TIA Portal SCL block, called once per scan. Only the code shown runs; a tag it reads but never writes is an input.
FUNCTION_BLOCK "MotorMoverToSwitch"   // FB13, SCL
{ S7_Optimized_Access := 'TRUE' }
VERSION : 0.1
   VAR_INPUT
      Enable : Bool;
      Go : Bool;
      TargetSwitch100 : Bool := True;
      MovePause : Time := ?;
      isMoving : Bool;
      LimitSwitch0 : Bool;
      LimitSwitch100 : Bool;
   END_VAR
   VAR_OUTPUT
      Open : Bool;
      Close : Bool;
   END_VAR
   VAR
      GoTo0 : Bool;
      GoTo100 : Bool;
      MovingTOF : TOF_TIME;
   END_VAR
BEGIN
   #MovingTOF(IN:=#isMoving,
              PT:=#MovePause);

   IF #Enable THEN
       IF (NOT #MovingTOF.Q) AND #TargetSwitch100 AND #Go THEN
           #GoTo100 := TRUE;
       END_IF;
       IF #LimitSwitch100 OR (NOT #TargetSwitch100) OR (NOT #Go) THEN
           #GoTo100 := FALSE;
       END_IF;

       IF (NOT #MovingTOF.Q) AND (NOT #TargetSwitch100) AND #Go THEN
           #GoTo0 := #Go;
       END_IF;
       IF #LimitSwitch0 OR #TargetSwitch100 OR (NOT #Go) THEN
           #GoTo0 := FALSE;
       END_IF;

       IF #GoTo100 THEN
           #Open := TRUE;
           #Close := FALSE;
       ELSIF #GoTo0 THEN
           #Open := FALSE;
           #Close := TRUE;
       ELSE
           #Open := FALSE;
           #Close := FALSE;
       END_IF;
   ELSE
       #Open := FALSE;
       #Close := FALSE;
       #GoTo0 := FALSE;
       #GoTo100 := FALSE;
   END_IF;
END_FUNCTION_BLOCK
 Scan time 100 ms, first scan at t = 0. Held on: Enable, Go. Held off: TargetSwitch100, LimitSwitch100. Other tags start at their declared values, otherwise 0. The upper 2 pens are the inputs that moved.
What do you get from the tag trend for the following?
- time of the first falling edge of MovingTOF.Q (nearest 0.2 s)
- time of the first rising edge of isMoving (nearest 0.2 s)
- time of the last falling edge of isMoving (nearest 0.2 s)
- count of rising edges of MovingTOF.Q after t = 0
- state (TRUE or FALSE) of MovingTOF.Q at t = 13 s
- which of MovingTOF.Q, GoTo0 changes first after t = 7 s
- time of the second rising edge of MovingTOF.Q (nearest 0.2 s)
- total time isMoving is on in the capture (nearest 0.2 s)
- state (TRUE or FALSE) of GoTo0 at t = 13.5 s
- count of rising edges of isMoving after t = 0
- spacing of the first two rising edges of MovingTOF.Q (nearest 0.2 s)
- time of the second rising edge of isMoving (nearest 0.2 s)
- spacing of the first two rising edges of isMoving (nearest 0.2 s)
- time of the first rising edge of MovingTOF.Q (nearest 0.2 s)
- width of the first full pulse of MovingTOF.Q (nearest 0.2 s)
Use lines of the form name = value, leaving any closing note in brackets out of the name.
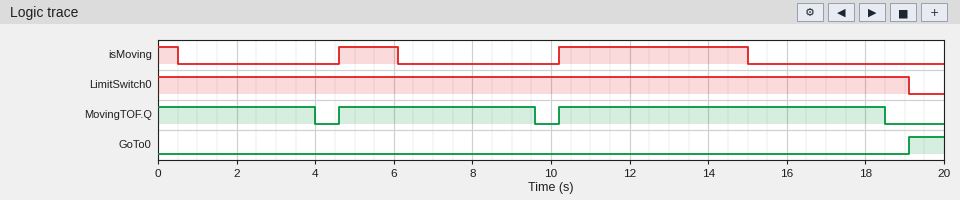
time of the first falling edge of MovingTOF.Q = 4.0 s
time of the first rising edge of isMoving = 4.6 s
time of the last falling edge of isMoving = 15.0 s
count of rising edges of MovingTOF.Q after t = 0 = 2
state (TRUE or FALSE) of MovingTOF.Q at t = 13 s = TRUE
which of MovingTOF.Q, GoTo0 changes first after t = 7 s = MovingTOF.Q
time of the second rising edge of MovingTOF.Q = 10.2 s
total time isMoving is on in the capture = 6.8 s
state (TRUE or FALSE) of GoTo0 at t = 13.5 s = FALSE
count of rising edges of isMoving after t = 0 = 2
spacing of the first two rising edges of MovingTOF.Q = 5.6 s
time of the second rising edge of isMoving = 10.2 s
spacing of the first two rising edges of isMoving = 5.6 s
time of the first rising edge of MovingTOF.Q = 4.6 s
width of the first full pulse of MovingTOF.Q = 5.0 s
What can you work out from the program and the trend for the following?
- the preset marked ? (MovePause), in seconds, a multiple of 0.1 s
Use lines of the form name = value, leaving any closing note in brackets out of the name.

the preset marked ? (MovePause), in seconds, a multiple of 0.1 s = 3.5 s
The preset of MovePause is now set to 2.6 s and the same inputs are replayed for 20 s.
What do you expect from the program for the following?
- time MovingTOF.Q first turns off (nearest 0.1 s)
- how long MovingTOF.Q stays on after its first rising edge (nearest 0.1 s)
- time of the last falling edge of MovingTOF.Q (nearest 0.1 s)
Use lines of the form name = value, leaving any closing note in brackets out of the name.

time MovingTOF.Q first turns off = 3.1 s
how long MovingTOF.Q stays on after its first rising edge = 4.1 s
time of the last falling edge of MovingTOF.Q = 17.6 s
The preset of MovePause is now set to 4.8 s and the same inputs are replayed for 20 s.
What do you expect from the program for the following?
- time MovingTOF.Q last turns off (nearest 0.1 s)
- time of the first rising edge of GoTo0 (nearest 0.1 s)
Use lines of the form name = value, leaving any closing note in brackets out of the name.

time MovingTOF.Q last turns off = 19.8 s
time of the first rising edge of GoTo0 = 19.8 s
